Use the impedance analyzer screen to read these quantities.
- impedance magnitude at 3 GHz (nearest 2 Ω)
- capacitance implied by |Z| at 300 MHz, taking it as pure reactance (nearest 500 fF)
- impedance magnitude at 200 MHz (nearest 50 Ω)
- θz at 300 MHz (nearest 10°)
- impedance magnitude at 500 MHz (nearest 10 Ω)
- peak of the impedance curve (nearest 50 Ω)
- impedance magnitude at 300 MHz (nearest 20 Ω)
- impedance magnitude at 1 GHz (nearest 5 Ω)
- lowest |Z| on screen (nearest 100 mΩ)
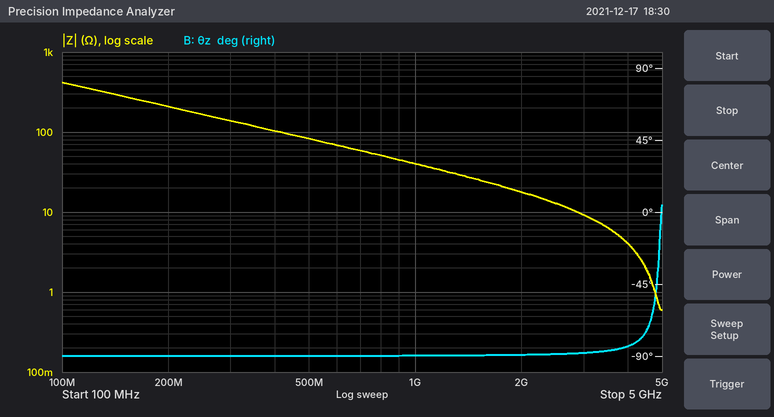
10 Ω
4.0 pF
200 Ω
-90°
80 Ω
400 Ω
140 Ω
40 Ω
600 mΩ
